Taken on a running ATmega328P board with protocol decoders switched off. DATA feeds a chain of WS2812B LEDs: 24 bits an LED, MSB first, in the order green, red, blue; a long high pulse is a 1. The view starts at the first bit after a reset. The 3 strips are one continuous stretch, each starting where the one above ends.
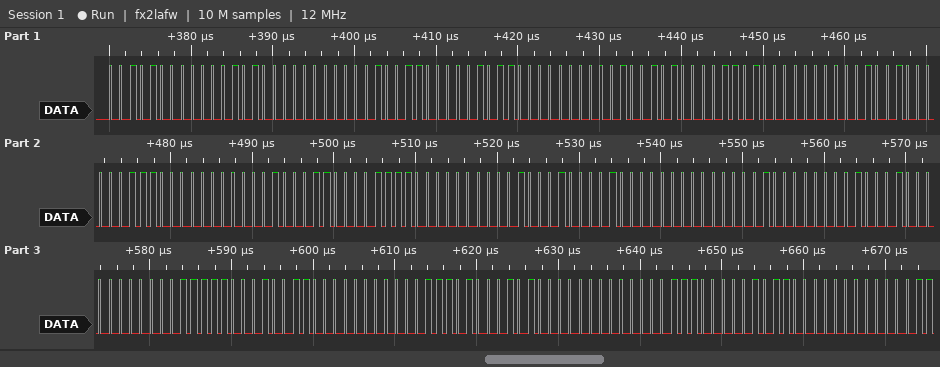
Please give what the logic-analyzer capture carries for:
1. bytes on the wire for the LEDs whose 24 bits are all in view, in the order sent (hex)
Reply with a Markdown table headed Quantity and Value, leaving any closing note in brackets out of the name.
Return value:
| Quantity | Value |
|---|---|
| bytes on the wire for the LEDs whose 24 bits are all in view, in the order sent | 28 0A 00 26 0B 00 25 0D 00 24 0E 00 23 0F 00 22 10 00 20 11 00 1F 13 00 1D 14 00 1C 16 00 |
